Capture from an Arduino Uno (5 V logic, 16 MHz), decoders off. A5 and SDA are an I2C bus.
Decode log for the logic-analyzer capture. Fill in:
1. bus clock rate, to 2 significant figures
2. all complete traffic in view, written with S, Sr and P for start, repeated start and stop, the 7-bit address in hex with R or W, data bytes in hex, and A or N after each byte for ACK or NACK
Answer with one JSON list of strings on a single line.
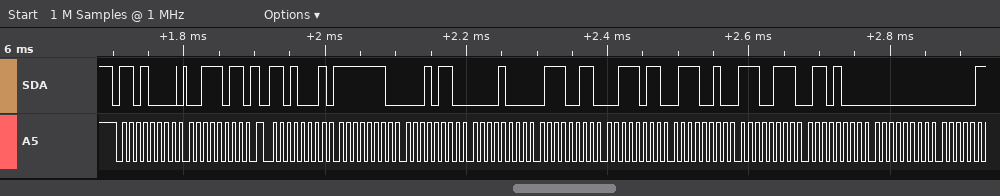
["100 kHz", "S 68W A 3B A Sr 68R A FE A 16 A 08 A 73 A 3B A 72 A E7 A 68 A 00 A"]
